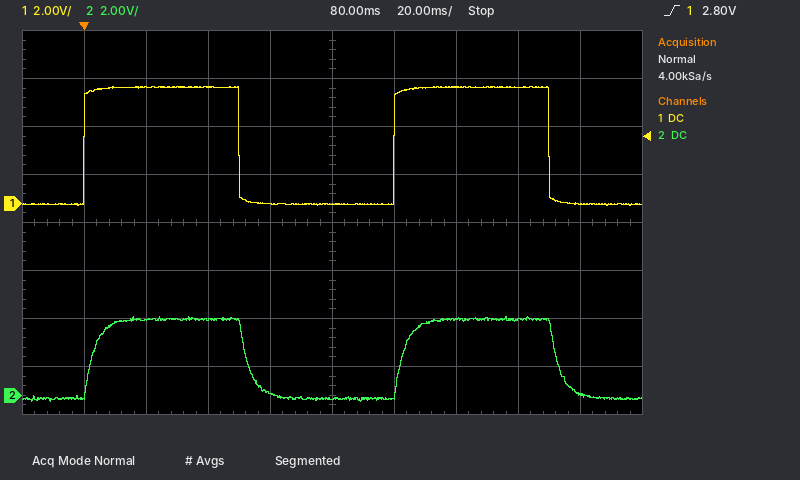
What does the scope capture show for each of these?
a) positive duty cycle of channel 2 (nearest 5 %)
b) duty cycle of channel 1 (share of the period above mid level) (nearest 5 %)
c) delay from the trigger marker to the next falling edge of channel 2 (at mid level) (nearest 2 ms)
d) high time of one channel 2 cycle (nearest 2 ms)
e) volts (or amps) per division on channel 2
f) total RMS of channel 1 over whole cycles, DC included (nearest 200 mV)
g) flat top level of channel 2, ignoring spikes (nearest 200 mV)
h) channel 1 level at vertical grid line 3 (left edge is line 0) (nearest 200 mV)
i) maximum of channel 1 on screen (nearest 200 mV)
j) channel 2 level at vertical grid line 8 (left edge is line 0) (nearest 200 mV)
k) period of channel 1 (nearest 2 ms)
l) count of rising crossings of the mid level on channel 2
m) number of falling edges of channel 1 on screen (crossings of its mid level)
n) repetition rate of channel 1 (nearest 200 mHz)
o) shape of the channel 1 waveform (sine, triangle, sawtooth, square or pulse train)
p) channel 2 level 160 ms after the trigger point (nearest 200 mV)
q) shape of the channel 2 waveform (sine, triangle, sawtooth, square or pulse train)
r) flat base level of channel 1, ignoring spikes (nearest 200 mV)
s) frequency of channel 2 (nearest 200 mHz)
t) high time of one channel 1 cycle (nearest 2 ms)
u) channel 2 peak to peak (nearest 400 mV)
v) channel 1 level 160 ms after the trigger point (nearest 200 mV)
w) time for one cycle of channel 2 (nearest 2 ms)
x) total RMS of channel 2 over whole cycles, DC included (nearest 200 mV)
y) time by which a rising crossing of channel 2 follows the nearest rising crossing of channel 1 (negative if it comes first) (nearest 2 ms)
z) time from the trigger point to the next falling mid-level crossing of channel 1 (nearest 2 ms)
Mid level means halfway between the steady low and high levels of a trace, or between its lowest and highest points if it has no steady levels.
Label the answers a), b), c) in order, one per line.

a) 50 %
b) 50 %
c) 52 ms
d) 50 ms
e) 2 V
f) 3.4 V
g) 3.2 V
h) 4.8 V
i) 4.8 V
j) 3.2 V
k) 100 ms
l) 2
m) 2
n) 10.0 Hz
o) square
p) 0.0 V
q) square
r) 0.0 V
s) 10.0 Hz
t) 50 ms
u) 3.6 V
v) 0.0 V
w) 100 ms
x) 2.2 V
y) +2 ms
z) 50 ms
